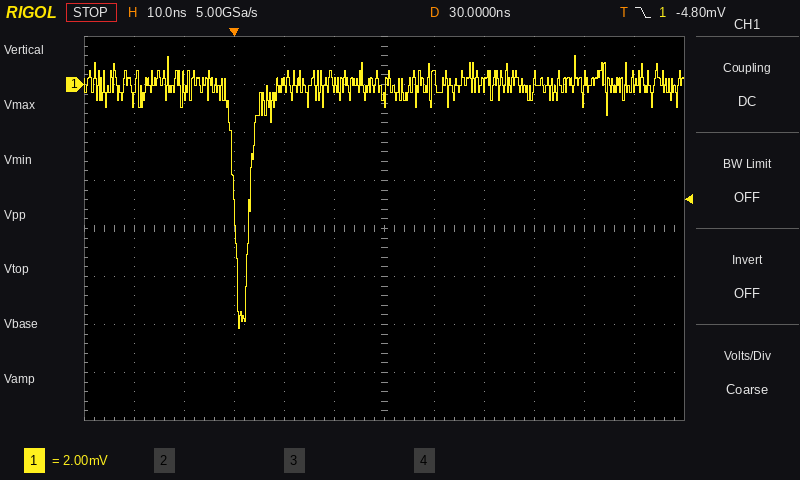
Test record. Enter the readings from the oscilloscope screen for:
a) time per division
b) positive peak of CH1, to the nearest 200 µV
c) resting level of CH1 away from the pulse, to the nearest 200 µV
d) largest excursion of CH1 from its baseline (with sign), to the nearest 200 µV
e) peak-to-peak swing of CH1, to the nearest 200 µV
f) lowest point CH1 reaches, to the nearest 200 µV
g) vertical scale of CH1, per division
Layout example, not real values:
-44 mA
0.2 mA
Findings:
10 ns
1.2 mV
0.0 mV
-10.2 mV
11.4 mV
-10.2 mV
2 mV
